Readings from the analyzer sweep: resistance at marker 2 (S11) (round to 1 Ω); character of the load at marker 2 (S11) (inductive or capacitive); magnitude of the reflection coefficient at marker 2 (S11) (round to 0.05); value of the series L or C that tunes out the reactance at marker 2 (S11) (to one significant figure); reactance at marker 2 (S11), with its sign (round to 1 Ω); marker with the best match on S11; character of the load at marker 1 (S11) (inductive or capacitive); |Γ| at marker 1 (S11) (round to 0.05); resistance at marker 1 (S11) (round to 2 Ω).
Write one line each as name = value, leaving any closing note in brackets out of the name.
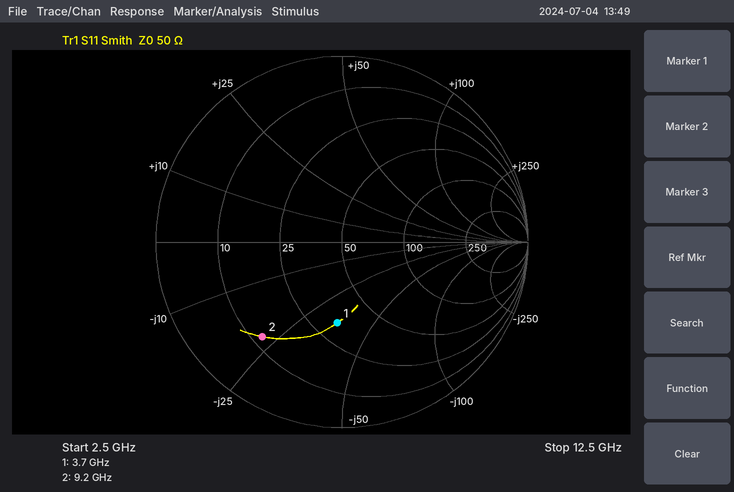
resistance at marker 2 (S11) = 12 Ω
character of the load at marker 2 (S11) = capacitive
magnitude of the reflection coefficient at marker 2 (S11) = 0.65
value of the series L or C that tunes out the reactance at marker 2 (S11) = 400 pH
reactance at marker 2 (S11), with its sign = -22 Ω
marker with the best match on S11 = marker 1
character of the load at marker 1 (S11) = capacitive
|Γ| at marker 1 (S11) = 0.45
resistance at marker 1 (S11) = 32 Ω
